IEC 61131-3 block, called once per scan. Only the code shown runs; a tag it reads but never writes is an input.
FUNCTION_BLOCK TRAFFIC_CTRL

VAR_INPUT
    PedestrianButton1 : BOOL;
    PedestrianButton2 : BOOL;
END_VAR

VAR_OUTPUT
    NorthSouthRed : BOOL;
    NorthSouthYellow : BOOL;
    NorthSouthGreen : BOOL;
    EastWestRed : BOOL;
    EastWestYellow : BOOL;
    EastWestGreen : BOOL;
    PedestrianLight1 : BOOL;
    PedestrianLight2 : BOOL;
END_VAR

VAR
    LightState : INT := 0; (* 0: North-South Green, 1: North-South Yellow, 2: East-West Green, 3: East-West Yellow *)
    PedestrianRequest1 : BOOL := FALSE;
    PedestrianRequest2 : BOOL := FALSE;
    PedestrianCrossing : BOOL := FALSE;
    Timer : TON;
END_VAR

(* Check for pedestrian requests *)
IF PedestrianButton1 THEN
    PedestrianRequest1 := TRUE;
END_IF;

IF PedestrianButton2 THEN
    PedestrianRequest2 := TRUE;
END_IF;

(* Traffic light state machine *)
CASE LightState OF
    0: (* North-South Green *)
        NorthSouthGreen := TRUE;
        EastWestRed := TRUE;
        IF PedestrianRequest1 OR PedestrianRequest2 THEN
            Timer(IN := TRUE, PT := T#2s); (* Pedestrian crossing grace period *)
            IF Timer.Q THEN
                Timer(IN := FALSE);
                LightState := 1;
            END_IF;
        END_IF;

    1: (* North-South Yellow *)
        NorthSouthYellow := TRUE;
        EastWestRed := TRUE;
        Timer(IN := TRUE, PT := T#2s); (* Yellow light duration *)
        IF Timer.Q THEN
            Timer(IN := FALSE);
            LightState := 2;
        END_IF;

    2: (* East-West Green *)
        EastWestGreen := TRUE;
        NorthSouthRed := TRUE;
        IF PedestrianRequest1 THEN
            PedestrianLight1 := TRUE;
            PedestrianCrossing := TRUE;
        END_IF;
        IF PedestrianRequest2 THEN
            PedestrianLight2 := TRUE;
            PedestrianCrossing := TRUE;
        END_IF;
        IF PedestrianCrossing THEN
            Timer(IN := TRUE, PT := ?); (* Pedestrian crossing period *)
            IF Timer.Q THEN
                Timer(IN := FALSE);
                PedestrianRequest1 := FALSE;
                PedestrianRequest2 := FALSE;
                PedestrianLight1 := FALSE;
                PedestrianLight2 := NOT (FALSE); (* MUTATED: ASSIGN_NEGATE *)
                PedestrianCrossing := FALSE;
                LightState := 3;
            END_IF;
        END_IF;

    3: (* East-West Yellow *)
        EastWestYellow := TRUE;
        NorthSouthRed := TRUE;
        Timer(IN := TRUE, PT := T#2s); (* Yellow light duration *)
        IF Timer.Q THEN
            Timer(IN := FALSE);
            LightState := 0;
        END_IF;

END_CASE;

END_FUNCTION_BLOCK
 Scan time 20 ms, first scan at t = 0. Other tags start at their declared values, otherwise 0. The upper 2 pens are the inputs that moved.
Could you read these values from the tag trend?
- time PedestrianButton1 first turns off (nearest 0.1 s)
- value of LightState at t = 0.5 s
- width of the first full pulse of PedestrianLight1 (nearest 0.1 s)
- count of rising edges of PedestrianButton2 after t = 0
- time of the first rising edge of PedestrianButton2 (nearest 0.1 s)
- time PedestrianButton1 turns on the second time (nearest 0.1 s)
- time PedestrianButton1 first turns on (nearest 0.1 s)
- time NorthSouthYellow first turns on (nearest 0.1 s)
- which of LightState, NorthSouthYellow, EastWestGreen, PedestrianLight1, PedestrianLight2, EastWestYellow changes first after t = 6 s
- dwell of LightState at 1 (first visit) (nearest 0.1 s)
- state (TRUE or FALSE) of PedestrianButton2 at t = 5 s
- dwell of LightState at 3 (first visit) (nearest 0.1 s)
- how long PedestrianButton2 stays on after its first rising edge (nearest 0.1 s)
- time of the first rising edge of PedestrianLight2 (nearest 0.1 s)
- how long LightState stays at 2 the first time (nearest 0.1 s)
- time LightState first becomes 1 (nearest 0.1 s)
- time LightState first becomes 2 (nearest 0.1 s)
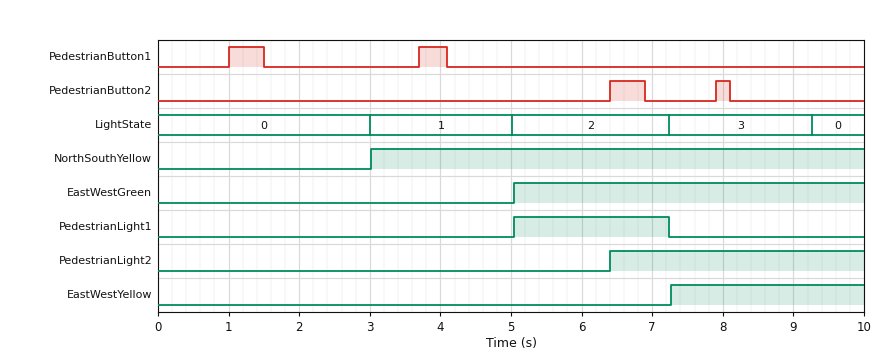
1.5 s
0
2.2 s
2
6.4 s
3.7 s
1.0 s
3.0 s
PedestrianLight2
2.0 s
FALSE
2.0 s
0.5 s
6.4 s
2.2 s
3.0 s
5.0 s
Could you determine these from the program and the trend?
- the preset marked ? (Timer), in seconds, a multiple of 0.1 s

2.2 s
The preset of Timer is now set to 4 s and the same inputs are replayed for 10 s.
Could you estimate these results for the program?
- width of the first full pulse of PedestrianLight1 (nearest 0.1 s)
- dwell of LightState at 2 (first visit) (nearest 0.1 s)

4.0 s
4.0 s
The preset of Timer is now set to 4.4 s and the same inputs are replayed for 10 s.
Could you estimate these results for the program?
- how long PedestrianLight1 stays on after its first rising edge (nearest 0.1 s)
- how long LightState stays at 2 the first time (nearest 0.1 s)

4.4 s
4.4 s
